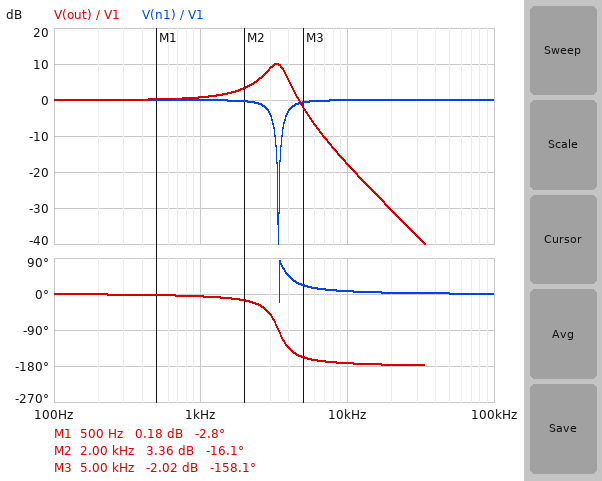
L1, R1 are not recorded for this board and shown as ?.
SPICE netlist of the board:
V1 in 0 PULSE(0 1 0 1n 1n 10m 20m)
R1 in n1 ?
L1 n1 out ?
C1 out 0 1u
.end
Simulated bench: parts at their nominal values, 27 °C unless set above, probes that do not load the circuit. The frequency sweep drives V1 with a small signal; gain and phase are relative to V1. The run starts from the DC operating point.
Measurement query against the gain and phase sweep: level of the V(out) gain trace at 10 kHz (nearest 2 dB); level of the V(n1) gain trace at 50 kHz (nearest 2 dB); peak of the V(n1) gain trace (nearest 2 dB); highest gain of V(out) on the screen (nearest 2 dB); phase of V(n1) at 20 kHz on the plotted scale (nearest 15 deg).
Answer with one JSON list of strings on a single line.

["-18 dB", "0 dB", "0 dB", "10 dB", "0 deg"]
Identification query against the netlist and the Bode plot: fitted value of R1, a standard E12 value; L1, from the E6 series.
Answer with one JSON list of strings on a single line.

["15 Ω", "2.2 mH"]
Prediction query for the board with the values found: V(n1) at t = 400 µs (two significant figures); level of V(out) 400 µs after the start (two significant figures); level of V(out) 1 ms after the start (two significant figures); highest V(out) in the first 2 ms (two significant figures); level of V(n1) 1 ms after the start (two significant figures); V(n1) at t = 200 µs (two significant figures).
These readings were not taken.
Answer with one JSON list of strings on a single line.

["930 mV", "1.1 V", "1.0 V", "1.6 V", "990 mV", "1.1 V"]
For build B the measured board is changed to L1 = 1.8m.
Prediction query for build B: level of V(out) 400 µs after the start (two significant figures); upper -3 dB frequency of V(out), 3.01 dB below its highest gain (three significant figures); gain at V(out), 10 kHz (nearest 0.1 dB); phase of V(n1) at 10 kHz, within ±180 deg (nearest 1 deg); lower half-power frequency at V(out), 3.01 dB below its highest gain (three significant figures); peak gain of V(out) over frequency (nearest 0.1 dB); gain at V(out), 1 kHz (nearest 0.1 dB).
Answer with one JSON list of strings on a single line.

["1.2 V", "4.25 kHz", "-15.8 dB", "9 deg", "2.88 kHz", "9.2 dB", "0.6 dB"]
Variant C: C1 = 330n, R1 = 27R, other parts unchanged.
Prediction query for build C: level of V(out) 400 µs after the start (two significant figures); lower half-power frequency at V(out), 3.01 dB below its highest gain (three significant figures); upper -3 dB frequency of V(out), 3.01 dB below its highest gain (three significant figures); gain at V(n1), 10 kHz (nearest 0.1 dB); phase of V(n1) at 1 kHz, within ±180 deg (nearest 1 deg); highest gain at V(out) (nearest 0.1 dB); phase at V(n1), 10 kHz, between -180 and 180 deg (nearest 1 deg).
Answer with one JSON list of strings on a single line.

["1.0 V", "4.65 kHz", "6.66 kHz", "-0.4 dB", "-3 deg", "9.7 dB", "17 deg"]
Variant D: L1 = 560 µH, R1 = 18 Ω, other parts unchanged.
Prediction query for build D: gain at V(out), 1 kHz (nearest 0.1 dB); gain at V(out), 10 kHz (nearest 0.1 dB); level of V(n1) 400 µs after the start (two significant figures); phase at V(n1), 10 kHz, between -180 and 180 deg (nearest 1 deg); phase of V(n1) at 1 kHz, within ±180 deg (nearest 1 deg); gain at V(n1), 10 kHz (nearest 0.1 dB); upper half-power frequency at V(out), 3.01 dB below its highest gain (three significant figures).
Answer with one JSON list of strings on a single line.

["0.1 dB", "-4.4 dB", "1.0 V", "43 deg", "-7 deg", "-2.7 dB", "8.00 kHz"]
